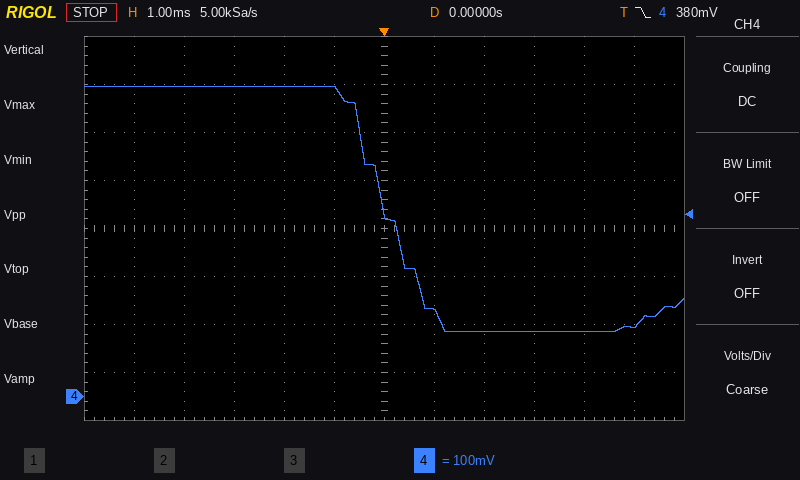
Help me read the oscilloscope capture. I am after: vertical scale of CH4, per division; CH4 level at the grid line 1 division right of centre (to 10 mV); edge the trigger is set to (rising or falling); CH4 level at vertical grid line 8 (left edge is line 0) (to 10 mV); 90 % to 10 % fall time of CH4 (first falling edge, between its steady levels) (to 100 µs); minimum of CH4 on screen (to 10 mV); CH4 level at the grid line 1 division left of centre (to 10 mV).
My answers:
100 mV
180 mV
falling
140 mV
1.4 ms
140 mV
640 mV
